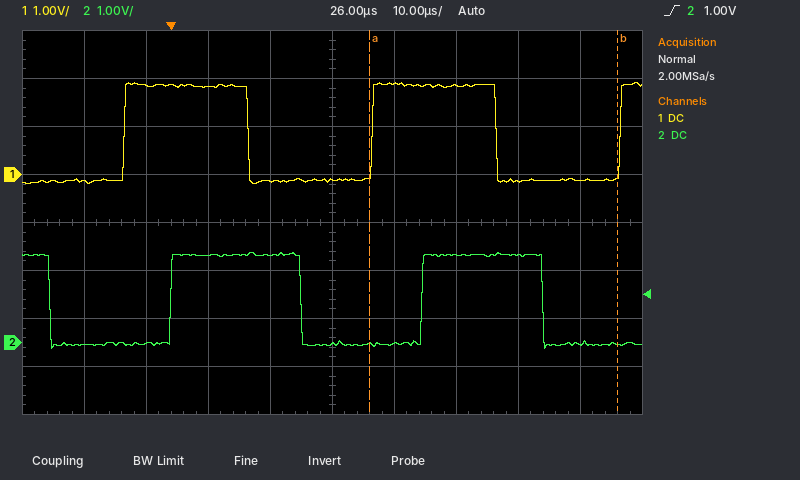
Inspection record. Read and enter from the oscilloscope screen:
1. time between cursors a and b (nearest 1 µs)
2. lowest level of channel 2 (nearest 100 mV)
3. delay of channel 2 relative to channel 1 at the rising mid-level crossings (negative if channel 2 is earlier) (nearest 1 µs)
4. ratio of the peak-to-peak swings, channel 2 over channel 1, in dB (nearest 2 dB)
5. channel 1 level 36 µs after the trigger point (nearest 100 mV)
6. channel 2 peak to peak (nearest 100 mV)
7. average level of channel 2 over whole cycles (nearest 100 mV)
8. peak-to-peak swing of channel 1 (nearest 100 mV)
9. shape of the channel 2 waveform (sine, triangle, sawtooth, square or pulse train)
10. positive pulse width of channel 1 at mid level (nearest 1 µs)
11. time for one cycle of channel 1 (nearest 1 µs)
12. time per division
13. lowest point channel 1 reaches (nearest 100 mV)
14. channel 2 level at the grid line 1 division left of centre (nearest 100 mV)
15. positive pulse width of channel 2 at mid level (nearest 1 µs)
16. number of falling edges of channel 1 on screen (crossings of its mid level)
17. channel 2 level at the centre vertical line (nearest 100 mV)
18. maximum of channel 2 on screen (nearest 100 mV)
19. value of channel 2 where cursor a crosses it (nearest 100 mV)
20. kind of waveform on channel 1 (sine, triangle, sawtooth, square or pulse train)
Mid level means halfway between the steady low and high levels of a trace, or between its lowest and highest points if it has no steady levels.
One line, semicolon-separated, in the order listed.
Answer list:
40 µs; -100 mV; +8 µs; 0 dB; 1.9 V; 2.0 V; 900 mV; 2.1 V; square; 20 µs; 40 µs; 10 µs; -200 mV; 1.8 V; 20 µs; 2; 0.0 V; 1.9 V; 0.0 V; square
